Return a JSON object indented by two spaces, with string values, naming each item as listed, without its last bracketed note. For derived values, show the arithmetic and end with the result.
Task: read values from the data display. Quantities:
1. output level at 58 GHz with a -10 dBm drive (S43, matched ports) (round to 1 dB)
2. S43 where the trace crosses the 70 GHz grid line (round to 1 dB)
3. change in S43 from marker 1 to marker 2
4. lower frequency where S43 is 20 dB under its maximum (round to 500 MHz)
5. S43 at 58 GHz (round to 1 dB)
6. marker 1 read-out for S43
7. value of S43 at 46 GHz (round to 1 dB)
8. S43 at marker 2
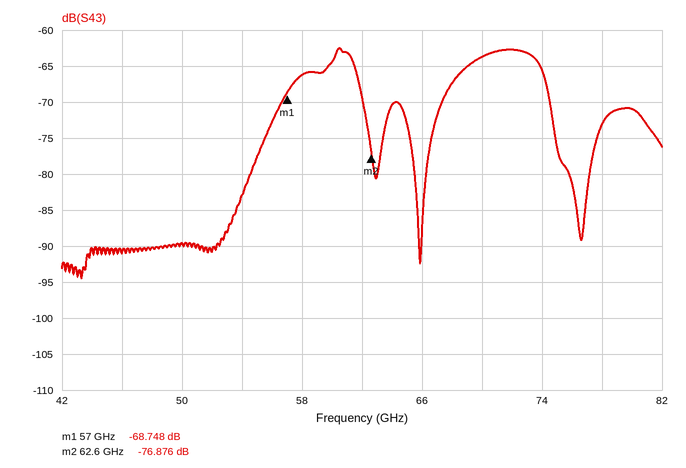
{
  "output level at 58 GHz with a -10 dBm drive (S43, matched ports)": "-10 dBm + (-66 dB) = -76 dBm",
  "S43 where the trace crosses the 70 GHz grid line": "-64 dB",
  "change in S43 from marker 1 to marker 2": "-76.876 − (-68.748) = -8.128 dB",
  "lower frequency where S43 is 20 dB under its maximum": "54.0 GHz",
  "S43 at 58 GHz": "-66 dB",
  "marker 1 read-out for S43": "-68.748 dB",
  "value of S43 at 46 GHz": "-91 dB",
  "S43 at marker 2": "-76.876 dB"
}
